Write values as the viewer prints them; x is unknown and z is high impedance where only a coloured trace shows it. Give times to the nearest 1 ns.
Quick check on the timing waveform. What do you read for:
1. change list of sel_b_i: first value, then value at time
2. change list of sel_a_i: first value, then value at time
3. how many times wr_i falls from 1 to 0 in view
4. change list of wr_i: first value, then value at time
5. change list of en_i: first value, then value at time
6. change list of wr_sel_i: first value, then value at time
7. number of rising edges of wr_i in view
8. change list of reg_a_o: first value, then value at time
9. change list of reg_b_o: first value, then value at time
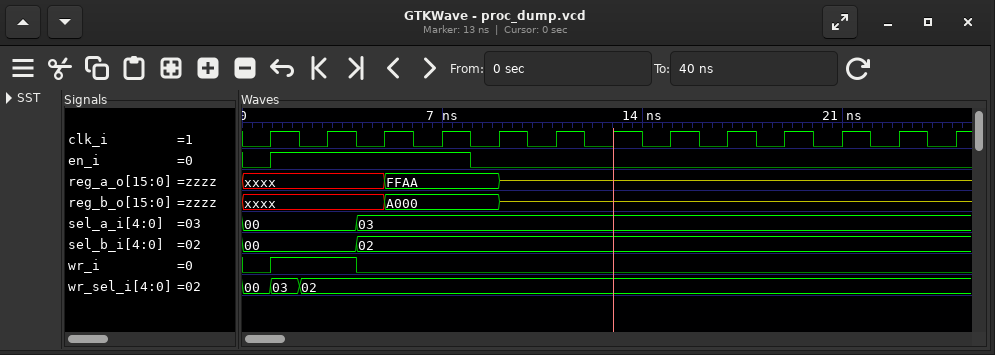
00, 02 at 4 ns
00, 03 at 4 ns
1
0, 1 at 1 ns, 0 at 4 ns
0, 1 at 1 ns, 0 at 8 ns
00, 03 at 1 ns, 02 at 2 ns
1
xxxx, FFAA at 5 ns, z at 9 ns
xxxx, A000 at 5 ns, z at 9 ns
